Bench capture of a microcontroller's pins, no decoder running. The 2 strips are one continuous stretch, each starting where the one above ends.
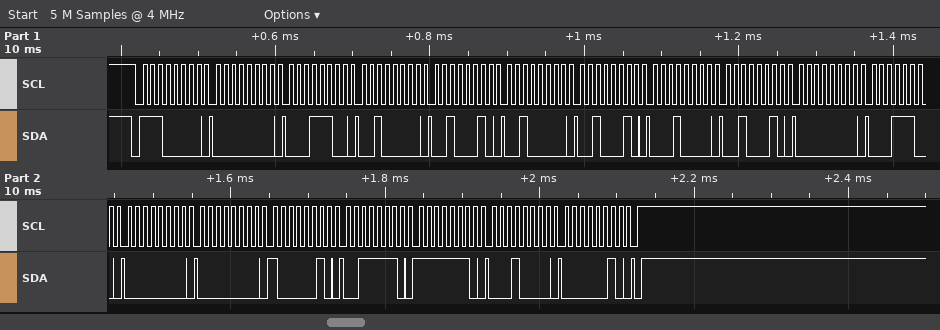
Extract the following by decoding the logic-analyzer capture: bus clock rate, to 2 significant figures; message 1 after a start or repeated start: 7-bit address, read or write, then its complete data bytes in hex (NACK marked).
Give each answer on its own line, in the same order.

100 kHz
0x70 write: 00 1C 20 22 20 22 10 22 00 1C 00 00 82 3E FE 10 02
